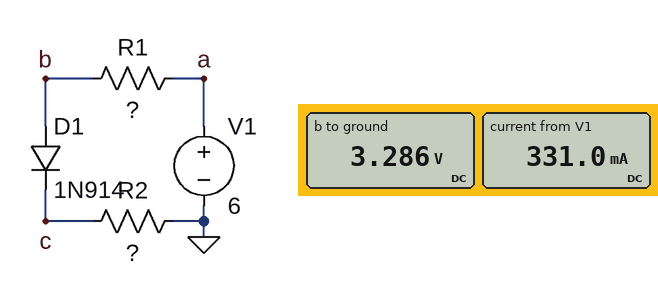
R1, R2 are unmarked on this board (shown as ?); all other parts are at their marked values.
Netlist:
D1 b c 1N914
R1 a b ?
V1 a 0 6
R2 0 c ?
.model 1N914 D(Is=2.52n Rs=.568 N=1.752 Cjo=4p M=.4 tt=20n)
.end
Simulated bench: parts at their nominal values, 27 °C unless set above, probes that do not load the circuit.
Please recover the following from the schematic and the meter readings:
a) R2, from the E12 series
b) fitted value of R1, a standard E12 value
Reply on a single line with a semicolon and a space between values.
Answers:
6.8 Ω; 8.2 Ω
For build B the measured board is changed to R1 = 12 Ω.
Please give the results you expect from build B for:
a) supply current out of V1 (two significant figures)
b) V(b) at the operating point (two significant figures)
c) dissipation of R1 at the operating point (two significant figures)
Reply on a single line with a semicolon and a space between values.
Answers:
270 mA; 2.8 V; 850 mW
